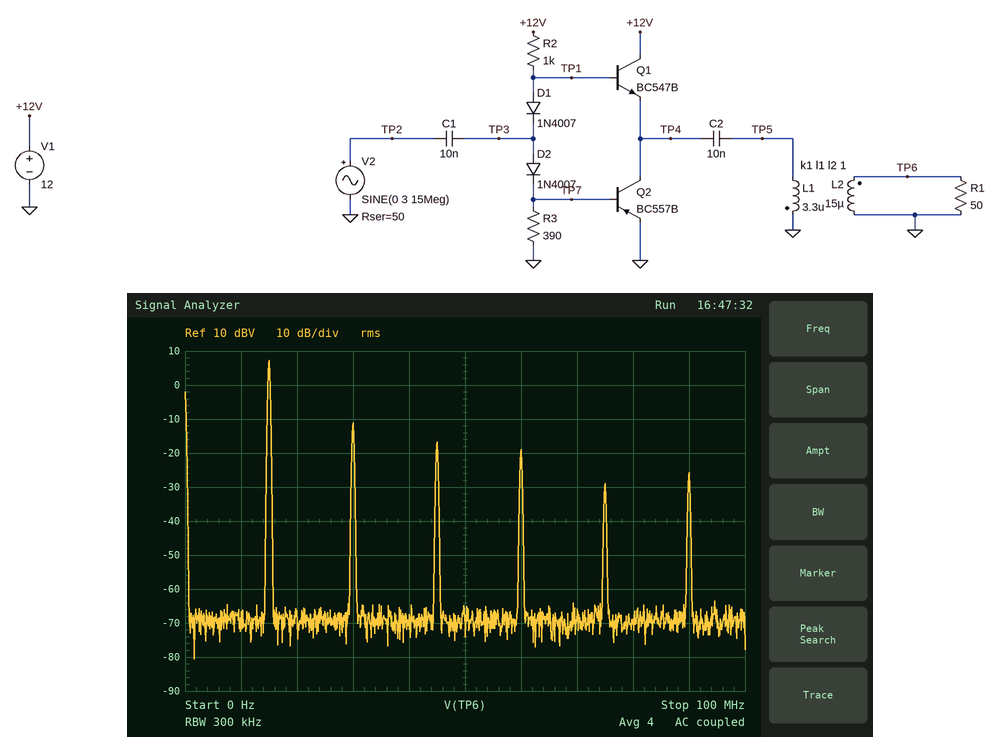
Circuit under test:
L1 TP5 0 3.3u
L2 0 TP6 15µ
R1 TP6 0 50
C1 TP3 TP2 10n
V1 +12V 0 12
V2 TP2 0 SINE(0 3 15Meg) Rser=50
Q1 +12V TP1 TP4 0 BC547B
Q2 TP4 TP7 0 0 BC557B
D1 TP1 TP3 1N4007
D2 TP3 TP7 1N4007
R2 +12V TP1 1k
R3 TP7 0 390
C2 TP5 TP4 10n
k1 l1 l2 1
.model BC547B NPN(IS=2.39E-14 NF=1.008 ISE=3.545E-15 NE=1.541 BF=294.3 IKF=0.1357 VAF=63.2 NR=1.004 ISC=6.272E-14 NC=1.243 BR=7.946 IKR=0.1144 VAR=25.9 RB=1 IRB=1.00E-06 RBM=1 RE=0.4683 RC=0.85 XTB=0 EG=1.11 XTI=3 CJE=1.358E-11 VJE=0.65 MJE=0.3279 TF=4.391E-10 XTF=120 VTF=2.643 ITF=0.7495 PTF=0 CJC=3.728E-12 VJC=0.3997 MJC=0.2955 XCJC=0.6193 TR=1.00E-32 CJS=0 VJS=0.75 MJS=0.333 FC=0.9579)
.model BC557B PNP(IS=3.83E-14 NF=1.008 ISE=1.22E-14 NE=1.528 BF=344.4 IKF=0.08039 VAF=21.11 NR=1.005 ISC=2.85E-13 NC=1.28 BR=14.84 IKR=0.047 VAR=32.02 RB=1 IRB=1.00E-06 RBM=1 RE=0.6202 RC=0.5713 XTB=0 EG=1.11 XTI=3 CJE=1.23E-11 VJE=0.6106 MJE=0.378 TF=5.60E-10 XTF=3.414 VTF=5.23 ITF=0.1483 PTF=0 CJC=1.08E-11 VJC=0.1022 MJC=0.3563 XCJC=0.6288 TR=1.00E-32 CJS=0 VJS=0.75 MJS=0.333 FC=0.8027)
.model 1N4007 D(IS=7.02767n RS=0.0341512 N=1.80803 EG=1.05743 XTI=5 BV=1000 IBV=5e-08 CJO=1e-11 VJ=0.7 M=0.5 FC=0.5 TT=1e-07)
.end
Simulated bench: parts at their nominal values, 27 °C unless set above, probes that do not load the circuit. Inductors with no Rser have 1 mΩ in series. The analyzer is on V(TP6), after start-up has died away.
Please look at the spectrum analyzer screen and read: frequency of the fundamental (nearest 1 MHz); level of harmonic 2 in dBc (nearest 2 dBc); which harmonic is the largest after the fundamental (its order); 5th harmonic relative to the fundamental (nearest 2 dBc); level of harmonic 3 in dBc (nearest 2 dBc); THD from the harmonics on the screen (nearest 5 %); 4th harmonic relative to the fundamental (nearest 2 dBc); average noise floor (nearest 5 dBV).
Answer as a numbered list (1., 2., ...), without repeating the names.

1. 15 MHz
2. -18 dBc
3. 2
4. -36 dBc
5. -24 dBc
6. 15 %
7. -26 dBc
8. -70 dBV
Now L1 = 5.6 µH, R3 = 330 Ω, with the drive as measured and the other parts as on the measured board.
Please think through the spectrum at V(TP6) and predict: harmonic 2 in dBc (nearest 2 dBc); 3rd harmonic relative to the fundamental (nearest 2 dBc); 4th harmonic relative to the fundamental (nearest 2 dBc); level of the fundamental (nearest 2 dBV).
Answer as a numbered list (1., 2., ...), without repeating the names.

1. -22 dBc
2. -36 dBc
3. -34 dBc
4. 6 dBV
